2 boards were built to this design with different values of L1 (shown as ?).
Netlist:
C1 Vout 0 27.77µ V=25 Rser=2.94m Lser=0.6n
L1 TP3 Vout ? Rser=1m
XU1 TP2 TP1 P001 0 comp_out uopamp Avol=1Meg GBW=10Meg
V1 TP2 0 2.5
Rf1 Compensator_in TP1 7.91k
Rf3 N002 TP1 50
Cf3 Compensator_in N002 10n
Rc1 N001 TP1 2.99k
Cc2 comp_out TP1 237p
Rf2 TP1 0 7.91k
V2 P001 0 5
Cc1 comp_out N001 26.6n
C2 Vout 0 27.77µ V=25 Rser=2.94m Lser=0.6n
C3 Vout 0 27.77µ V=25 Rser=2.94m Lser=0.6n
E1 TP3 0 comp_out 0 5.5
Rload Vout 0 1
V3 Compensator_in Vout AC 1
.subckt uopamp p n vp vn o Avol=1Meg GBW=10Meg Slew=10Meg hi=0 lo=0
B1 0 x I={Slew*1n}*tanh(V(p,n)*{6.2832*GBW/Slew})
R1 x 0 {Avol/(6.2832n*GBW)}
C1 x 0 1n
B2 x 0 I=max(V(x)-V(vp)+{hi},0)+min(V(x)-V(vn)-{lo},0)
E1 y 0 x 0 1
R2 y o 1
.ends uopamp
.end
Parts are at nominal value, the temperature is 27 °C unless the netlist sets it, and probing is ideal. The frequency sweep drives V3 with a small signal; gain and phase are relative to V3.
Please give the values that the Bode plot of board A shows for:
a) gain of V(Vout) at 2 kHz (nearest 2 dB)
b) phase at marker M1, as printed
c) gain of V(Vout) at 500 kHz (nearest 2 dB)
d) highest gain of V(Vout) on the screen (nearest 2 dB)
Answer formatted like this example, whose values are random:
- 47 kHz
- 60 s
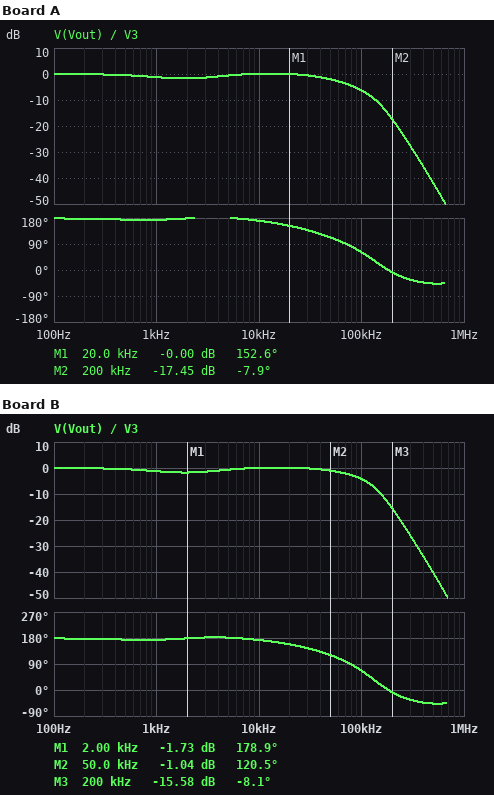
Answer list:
- -2 dB
- 152.6 deg
- -42 dB
- 0 dB
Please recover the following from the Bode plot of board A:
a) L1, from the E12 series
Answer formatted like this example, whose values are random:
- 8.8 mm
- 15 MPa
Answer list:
- 8.2 µH
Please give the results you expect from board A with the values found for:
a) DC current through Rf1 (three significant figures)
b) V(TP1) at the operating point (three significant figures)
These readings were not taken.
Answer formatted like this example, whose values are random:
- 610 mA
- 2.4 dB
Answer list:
- 316 µA
- 2.50 V
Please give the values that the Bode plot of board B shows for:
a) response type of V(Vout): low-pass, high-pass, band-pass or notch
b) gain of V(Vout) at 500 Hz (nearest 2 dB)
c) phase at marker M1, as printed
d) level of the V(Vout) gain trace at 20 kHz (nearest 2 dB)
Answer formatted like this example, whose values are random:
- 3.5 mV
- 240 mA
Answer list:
- low-pass
- 0 dB
- 178.9 deg
- 0 dB
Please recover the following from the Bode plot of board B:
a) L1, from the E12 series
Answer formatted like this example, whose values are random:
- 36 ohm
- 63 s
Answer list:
- 6.8 µH
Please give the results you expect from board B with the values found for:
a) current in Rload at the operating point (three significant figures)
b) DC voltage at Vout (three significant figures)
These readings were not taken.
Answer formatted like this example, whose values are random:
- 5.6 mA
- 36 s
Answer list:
- 5.00 A
- 5.00 V
